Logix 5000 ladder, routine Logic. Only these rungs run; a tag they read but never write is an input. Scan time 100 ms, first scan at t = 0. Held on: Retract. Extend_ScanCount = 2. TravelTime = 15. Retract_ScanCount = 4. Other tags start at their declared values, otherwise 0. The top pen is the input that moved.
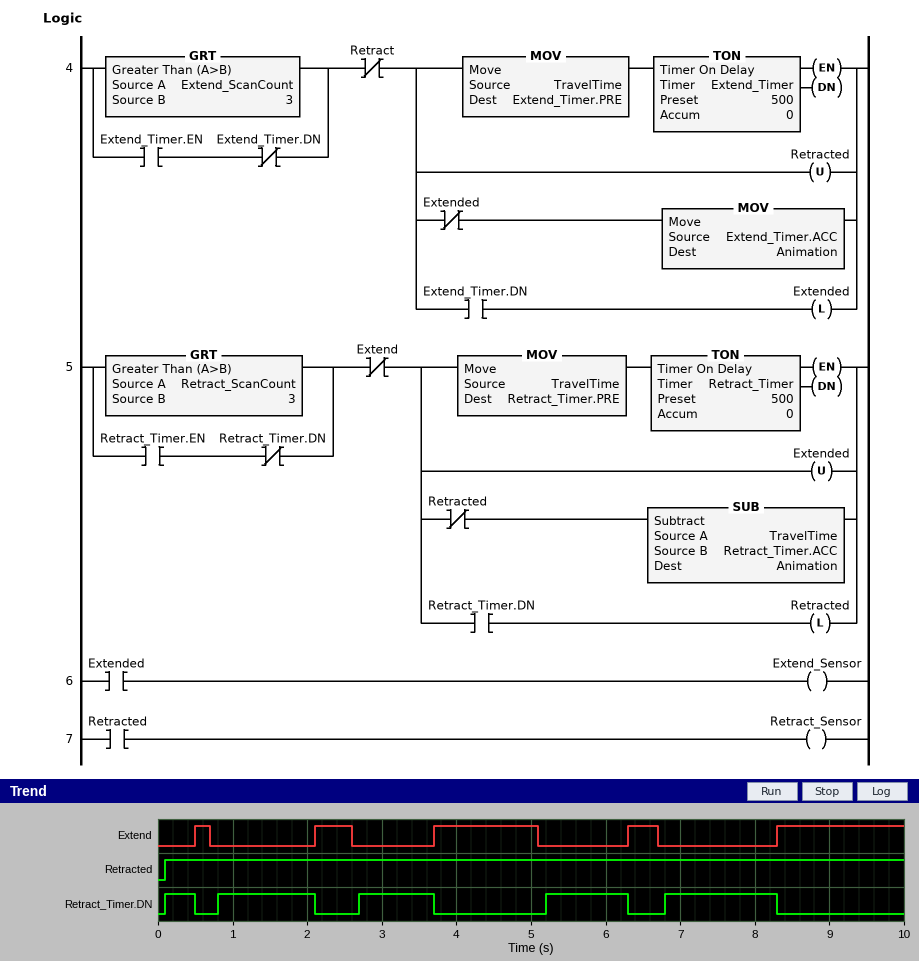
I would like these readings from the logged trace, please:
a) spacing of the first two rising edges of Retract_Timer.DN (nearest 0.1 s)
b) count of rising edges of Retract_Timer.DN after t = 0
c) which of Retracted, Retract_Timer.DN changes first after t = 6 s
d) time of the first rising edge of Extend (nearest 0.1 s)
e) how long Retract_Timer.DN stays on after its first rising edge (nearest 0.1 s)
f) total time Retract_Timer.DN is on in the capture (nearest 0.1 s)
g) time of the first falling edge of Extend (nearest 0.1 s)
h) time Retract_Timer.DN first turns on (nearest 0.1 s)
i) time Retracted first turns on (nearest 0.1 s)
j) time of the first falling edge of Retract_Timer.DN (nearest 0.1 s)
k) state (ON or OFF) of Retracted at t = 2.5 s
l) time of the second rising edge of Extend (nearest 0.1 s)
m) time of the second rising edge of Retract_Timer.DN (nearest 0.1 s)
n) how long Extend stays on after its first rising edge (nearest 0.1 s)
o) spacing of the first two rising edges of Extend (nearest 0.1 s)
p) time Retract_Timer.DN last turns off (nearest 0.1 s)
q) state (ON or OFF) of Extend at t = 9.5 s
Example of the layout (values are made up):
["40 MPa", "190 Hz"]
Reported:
["0.7 s", "5", "Retract_Timer.DN", "0.5 s", "0.4 s", "5.3 s", "0.7 s", "0.1 s", "0.1 s", "0.5 s", "ON", "2.1 s", "0.8 s", "0.2 s", "1.6 s", "8.3 s", "ON"]
